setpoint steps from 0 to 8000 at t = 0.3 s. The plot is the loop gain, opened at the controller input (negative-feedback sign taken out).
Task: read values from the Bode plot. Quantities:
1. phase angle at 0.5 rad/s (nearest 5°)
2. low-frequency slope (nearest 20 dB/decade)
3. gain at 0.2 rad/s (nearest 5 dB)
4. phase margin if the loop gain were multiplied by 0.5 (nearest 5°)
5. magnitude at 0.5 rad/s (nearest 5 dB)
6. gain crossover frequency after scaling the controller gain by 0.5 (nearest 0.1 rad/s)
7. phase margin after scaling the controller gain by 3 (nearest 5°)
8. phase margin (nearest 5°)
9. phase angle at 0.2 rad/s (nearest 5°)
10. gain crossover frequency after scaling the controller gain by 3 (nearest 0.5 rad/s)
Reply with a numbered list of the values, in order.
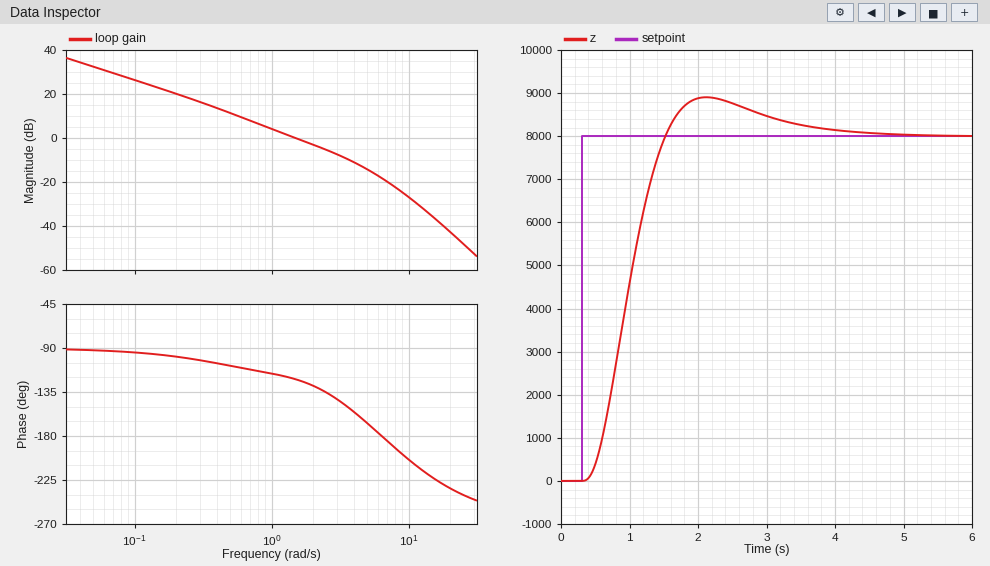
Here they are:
1. -110°
2. -20 dB/decade
3. 20 dB
4. 65°
5. 10 dB
6. 0.8 rad/s
7. 30°
8. 60°
9. -100°
10. 3.5 rad/s
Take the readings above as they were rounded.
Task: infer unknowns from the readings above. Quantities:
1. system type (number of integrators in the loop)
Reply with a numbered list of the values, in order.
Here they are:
1. 1
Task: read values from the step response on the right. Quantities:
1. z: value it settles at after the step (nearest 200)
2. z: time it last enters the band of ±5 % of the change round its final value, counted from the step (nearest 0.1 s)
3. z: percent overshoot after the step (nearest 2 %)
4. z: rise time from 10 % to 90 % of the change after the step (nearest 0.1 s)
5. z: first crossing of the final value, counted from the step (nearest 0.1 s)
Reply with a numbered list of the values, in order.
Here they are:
1. 8000
2. 2.8 s
3. 12 %
4. 0.8 s
5. 1.2 s
